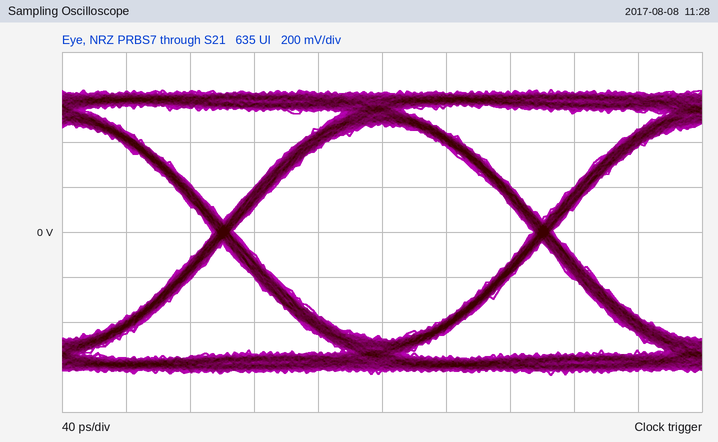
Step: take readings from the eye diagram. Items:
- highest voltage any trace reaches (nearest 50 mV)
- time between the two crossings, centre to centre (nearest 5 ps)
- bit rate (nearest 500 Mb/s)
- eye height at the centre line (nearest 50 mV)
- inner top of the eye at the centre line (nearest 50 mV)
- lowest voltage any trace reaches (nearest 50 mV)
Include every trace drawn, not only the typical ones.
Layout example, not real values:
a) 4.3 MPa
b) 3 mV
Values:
a) 650 mV
b) 200 ps
c) 5.0 Gb/s
d) 950 mV
e) 500 mV
f) -650 mV
